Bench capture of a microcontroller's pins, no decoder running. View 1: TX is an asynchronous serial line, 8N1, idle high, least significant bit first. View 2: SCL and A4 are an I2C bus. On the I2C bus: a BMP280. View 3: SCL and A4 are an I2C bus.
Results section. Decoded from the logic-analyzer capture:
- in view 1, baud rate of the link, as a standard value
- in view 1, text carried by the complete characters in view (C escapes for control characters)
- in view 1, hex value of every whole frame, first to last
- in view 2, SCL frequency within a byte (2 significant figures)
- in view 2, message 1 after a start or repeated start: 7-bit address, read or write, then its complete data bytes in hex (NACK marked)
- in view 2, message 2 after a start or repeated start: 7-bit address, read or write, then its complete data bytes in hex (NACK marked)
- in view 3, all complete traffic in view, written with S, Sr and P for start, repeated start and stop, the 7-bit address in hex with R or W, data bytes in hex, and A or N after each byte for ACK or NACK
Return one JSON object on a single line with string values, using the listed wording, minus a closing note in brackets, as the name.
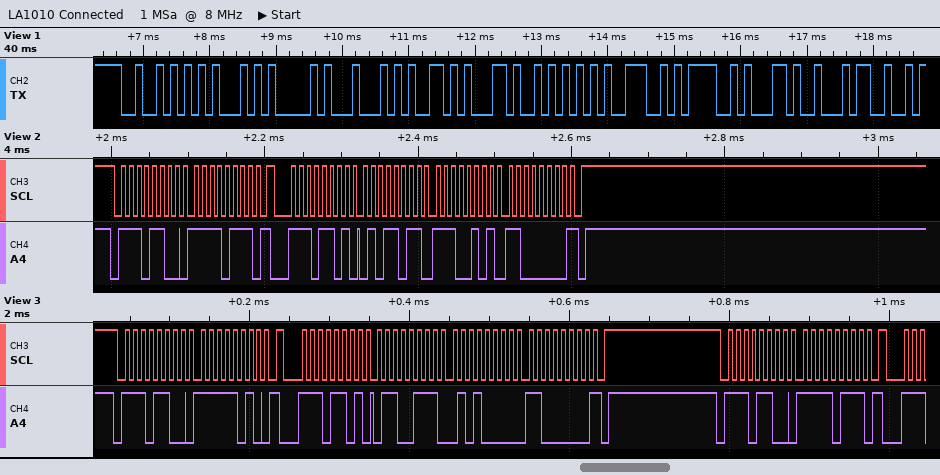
{"in view 1, baud rate of the link, as a standard value": "9600 baud", "in view 1, text carried by the complete characters in view": "\"READY,UNO,4\"", "in view 1, hex value of every whole frame, first to last": "52 45 41 44 59 2C 55 4E 4F 2C 34", "in view 2, SCL frequency within a byte": "100 kHz", "in view 2, message 1 after a start or repeated start: 7-bit address, read or write, then its complete data bytes in hex": "0x76 write: F7", "in view 2, message 2 after a start or repeated start: 7-bit address, read or write, then its complete data bytes in hex": "0x76 read: 5B E5 C0 NACK", "in view 3, all complete traffic in view, written with S, Sr and P for start, repeated start and stop, the 7-bit address in hex with R or W, data bytes in hex, and A or N after each byte for ACK or NACK": "S 76W A FA A Sr 76R A 67 A 50 A C0 N P S 76W A F7 A"}
